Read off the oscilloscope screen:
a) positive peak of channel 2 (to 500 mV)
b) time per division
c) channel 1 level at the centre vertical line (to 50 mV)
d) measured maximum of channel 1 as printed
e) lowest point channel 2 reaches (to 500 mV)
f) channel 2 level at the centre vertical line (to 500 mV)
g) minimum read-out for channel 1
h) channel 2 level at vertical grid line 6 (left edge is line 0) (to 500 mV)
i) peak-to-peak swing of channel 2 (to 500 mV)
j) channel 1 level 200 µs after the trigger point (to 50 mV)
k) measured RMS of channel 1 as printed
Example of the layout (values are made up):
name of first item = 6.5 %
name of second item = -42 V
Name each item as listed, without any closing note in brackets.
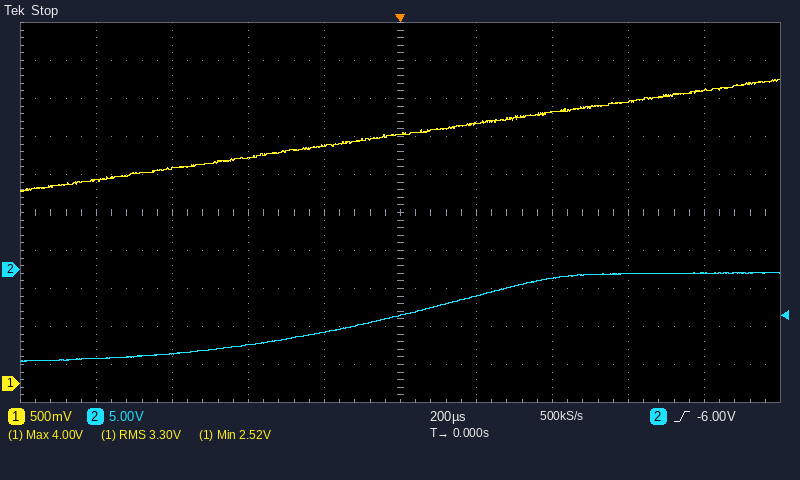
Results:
positive peak of channel 2 = -500 mV
time per division = 200 µs
channel 1 level at the centre vertical line = 3.30 V
measured maximum of channel 1 as printed = 4.00 V
lowest point channel 2 reaches = -12.0 V
channel 2 level at the centre vertical line = -6.0 V
minimum read-out for channel 1 = 2.52 V
channel 2 level at vertical grid line 6 (left edge is line 0) = -3.5 V
peak-to-peak swing of channel 2 = 11.5 V
channel 1 level 200 µs after the trigger point = 3.40 V
measured RMS of channel 1 as printed = 3.30 V
